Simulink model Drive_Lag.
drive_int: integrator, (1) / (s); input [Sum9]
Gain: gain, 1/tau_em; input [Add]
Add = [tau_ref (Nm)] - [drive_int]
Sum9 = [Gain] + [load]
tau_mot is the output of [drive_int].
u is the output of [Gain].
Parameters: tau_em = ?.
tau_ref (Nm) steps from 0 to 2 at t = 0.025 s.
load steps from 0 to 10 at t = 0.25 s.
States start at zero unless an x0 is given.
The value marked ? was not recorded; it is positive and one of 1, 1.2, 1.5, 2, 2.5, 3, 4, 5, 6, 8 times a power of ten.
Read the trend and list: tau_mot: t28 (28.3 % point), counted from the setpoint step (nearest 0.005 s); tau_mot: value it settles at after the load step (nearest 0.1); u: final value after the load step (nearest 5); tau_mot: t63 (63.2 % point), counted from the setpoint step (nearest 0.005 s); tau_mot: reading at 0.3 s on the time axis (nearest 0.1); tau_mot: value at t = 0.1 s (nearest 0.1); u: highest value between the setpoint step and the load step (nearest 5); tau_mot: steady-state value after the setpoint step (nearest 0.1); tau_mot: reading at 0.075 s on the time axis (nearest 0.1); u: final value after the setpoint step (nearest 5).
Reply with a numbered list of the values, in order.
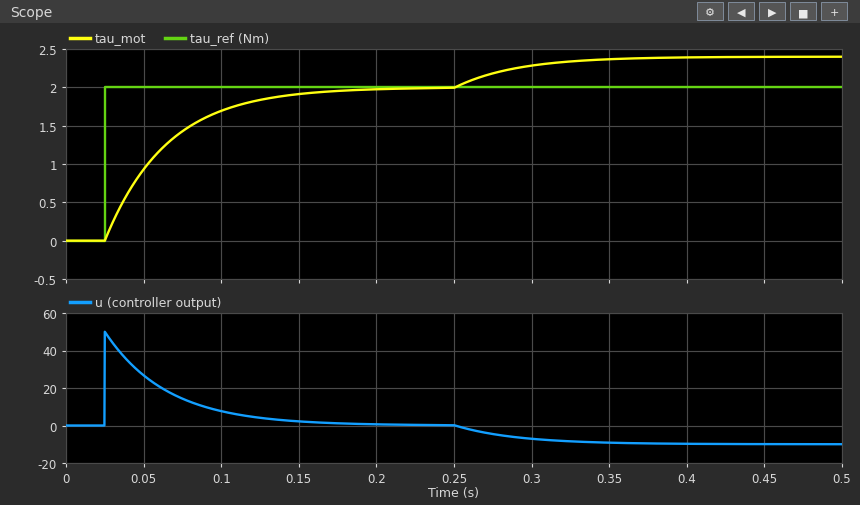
1. 0.015 s
2. 2.4
3. -10
4. 0.040 s
5. 2.3
6. 1.7
7. 50
8. 2.0
9. 1.4
10. 0
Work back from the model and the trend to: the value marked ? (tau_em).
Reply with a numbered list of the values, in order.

1. 0.04
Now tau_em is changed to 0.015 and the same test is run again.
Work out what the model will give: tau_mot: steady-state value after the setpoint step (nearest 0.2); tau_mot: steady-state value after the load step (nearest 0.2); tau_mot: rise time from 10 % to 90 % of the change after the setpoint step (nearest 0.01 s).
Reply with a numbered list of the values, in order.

1. 2.0
2. 2.2
3. 0.03 s
